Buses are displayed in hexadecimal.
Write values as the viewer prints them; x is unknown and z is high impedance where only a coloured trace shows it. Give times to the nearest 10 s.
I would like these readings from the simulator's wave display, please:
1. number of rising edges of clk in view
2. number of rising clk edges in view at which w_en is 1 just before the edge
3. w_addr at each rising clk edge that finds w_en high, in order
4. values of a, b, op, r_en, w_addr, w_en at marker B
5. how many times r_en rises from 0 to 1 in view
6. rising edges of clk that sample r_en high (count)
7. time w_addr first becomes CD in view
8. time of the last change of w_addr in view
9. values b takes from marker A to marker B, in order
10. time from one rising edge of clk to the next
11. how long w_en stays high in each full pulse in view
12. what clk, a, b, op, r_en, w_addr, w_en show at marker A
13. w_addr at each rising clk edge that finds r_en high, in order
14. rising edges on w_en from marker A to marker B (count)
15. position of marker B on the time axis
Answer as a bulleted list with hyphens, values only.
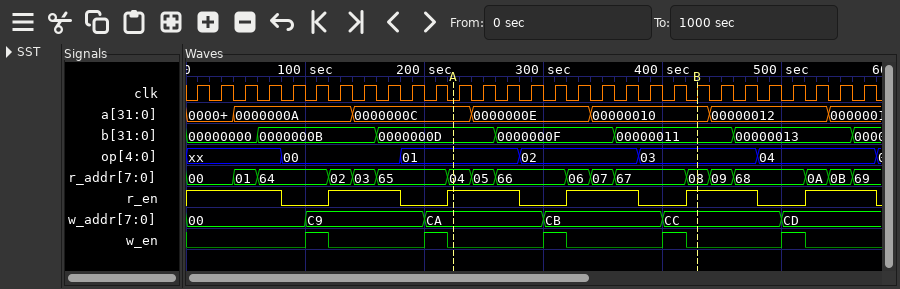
- 29
- 5
- C9, CA, CB, CC, CD
- a=00000010, b=00000011, op=03, r_en=1, w_addr=CC, w_en=0
- 5
- 19
- 500 s
- 500 s
- 0000000D, 0000000F, 00000011
- 20 s
- 20 s, 20 s, 20 s, 20 s, 20 s
- clk=0, a=0000000C, b=0000000D, op=01, r_en=1, w_addr=CA, w_en=0
- 00, 00, 00, 00, C9, C9, C9, CA, CA, CA, CB, CB, CB, CC, CC, CC, CD, CD, CD
- 2
- 430 s
